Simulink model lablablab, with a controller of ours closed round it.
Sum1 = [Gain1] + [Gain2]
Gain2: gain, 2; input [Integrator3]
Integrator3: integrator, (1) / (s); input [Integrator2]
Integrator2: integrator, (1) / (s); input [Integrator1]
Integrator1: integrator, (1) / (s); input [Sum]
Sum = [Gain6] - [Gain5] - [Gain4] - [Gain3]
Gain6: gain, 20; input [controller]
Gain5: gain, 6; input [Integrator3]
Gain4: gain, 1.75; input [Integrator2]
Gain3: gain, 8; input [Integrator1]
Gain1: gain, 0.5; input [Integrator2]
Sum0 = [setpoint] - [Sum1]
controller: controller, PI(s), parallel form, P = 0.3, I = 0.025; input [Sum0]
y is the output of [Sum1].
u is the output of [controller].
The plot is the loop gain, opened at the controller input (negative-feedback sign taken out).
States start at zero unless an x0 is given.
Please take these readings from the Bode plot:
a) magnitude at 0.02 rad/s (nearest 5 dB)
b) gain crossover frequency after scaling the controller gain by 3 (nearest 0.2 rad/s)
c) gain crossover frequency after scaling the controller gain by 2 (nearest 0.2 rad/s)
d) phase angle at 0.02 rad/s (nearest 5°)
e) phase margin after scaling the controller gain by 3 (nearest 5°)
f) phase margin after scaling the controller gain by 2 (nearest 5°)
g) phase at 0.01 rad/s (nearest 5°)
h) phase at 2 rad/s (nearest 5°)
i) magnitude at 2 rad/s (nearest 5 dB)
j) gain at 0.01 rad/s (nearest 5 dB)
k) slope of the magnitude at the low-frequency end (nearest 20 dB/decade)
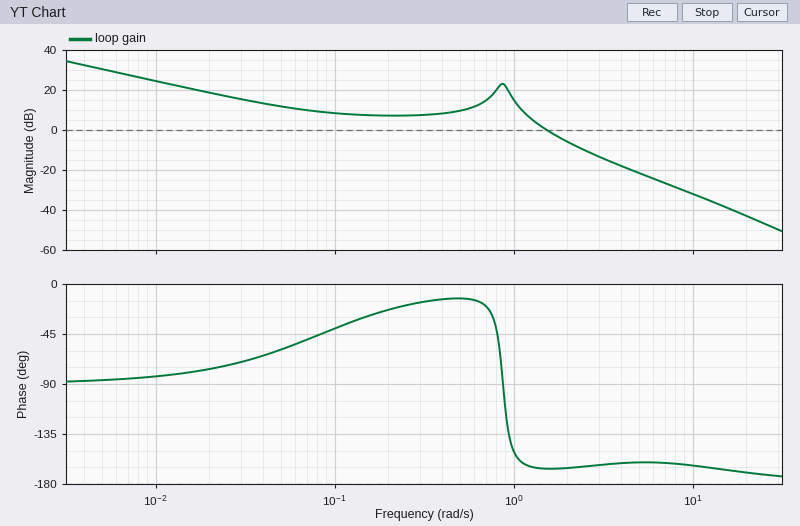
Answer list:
20 dB
2.4 rad/s
2.0 rad/s
-75°
15°
15°
-85°
-165°
-5 dB
25 dB
-20 dB/decade
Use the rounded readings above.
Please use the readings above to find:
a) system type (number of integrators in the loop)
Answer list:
1
